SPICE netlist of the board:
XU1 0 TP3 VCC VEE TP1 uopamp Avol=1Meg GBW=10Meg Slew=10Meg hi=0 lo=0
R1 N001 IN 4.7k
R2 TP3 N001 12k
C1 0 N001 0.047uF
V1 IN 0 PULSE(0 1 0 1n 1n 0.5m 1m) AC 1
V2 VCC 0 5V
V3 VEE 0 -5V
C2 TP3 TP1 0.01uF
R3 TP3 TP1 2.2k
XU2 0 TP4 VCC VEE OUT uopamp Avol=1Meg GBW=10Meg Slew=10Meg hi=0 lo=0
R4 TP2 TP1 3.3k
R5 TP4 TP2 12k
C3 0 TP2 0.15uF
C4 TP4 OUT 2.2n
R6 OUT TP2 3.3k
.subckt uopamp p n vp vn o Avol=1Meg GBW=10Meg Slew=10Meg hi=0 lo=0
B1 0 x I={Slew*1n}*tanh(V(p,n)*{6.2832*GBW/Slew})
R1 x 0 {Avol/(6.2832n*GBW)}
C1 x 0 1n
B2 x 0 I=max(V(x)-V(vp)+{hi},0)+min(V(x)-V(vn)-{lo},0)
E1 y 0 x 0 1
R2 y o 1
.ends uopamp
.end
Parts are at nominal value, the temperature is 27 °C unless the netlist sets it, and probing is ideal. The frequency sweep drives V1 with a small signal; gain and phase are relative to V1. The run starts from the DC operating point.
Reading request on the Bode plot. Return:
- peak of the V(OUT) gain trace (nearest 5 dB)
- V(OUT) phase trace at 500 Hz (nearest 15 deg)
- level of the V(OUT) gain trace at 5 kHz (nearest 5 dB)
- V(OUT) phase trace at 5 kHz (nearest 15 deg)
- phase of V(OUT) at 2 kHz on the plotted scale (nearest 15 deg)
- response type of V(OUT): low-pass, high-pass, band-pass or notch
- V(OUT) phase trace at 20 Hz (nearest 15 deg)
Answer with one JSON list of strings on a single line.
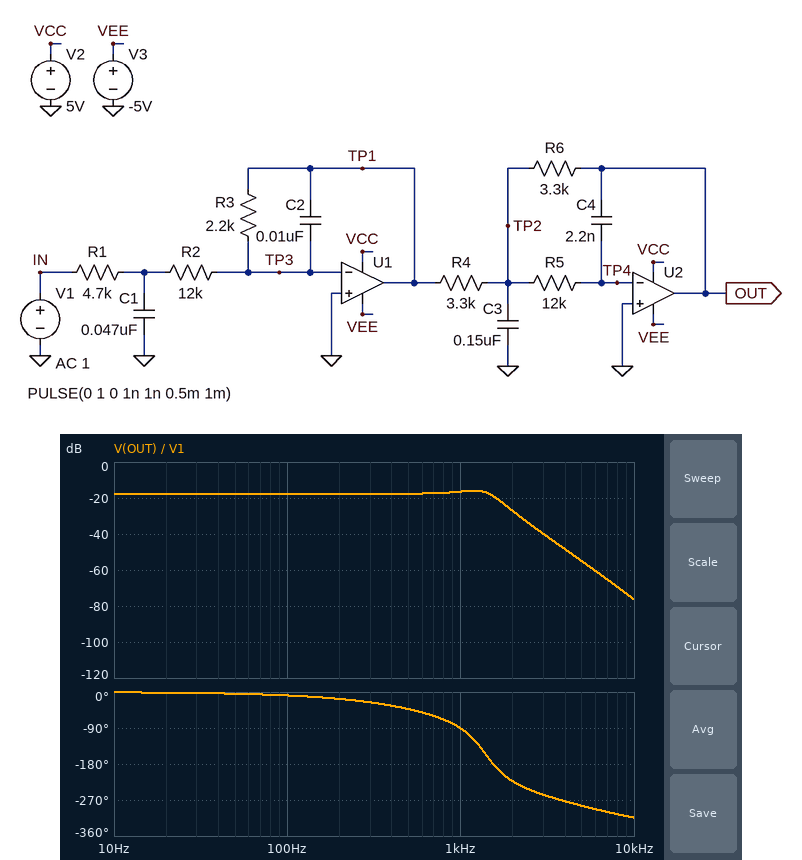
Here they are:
["-15 dB", "-45 deg", "-55 dB", "-285 deg", "-225 deg", "low-pass", "0 deg"]
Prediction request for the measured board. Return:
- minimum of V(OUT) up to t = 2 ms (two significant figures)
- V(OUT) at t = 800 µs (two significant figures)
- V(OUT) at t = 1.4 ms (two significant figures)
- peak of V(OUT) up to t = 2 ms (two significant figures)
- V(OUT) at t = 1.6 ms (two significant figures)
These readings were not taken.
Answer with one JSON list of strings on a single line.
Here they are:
["-29 mV", "41 mV", "140 mV", "160 mV", "150 mV"]
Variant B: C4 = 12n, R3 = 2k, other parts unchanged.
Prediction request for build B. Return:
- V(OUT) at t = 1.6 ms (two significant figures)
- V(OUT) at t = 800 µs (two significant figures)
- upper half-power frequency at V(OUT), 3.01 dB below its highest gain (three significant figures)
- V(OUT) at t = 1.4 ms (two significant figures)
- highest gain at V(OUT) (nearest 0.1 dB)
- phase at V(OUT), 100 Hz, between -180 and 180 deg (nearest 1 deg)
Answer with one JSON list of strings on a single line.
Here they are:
["71 mV", "84 mV", "589 Hz", "49 mV", "-18.4 dB", "-18 deg"]
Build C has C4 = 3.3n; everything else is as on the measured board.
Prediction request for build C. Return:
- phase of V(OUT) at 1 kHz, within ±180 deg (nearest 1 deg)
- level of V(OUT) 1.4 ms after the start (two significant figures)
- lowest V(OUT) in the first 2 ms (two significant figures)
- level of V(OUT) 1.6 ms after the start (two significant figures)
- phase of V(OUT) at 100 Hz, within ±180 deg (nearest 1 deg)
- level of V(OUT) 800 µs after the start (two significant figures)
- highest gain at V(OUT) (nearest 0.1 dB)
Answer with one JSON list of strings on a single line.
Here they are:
["-121 deg", "100 mV", "-27 mV", "160 mV", "-10 deg", "83 mV", "-16.2 dB"]
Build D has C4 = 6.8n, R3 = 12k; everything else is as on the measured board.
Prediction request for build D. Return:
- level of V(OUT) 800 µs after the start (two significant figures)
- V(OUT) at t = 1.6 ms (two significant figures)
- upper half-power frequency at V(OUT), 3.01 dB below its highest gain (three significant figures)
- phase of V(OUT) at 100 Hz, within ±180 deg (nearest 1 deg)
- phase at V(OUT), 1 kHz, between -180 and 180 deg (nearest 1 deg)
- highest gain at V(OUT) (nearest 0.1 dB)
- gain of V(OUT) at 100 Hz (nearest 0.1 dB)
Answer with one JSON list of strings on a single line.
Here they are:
["610 mV", "410 mV", "801 Hz", "-17 deg", "161 deg", "-2.8 dB", "-2.9 dB"]
